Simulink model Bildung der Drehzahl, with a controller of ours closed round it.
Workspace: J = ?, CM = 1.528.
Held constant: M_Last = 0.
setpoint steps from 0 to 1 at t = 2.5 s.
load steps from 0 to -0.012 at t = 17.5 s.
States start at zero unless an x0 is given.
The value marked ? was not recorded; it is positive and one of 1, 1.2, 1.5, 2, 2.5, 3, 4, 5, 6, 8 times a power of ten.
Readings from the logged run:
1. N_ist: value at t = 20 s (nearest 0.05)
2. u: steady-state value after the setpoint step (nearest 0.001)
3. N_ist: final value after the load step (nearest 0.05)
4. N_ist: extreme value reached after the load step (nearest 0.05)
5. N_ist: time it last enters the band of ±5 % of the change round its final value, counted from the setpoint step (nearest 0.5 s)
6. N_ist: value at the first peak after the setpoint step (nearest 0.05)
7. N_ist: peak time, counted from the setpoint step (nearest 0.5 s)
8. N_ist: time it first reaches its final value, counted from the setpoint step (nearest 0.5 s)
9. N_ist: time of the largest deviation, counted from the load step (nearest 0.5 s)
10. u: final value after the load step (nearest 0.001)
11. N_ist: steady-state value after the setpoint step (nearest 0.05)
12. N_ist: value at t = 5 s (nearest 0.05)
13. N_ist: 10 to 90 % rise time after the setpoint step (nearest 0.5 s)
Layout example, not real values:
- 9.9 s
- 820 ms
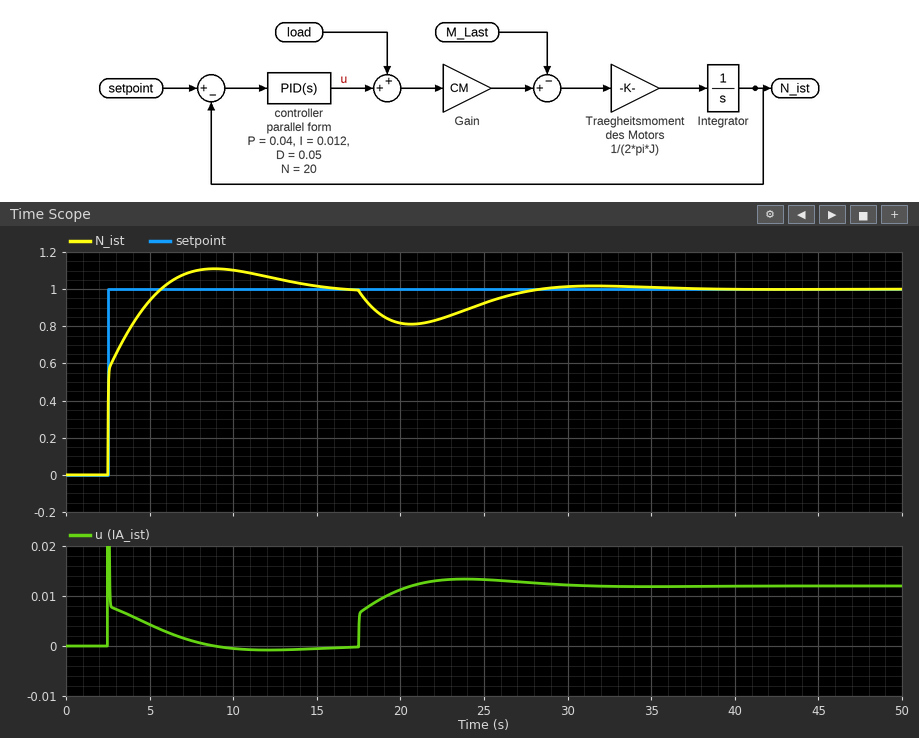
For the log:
- 0.80
- 0.000
- 1.00
- 0.80
- 10.5 s
- 1.10
- 6.5 s
- 3.0 s
- 3.0 s
- 0.012
- 1.00
- 0.95
- 2.0 s
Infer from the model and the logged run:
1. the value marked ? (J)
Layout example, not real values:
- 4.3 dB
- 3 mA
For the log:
- 0.01
